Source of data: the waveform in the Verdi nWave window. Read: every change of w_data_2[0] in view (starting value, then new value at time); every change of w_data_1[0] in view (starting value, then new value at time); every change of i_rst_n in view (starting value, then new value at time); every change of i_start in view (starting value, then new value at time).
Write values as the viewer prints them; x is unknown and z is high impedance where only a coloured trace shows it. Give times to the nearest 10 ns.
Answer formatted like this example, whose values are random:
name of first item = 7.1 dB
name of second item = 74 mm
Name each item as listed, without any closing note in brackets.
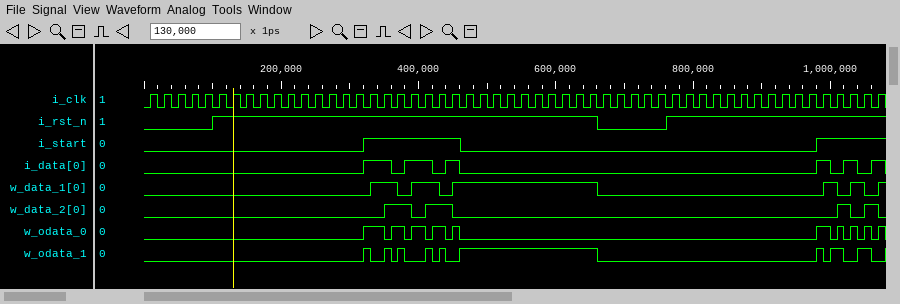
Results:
every change of w_data_2[0] in view = 0, 1 at 350 ns, 0 at 390 ns, 1 at 410 ns, 0 at 450 ns, 1 at 1010 ns, 0 at 1030 ns, 1 at 1050 ns, 0 at 1070 ns
every change of w_data_1[0] in view = 0, 1 at 330 ns, 0 at 370 ns, 1 at 390 ns, 0 at 430 ns, 1 at 450 ns, 0 at 660 ns, 1 at 990 ns, 0 at 1010 ns, 1 at 1030 ns, 0 at 1050 ns, 1 at 1070 ns
every change of i_rst_n in view = 0, 1 at 100 ns, 0 at 660 ns, 1 at 760 ns
every change of i_start in view = 0, 1 at 320 ns, 0 at 460 ns, 1 at 980 ns
